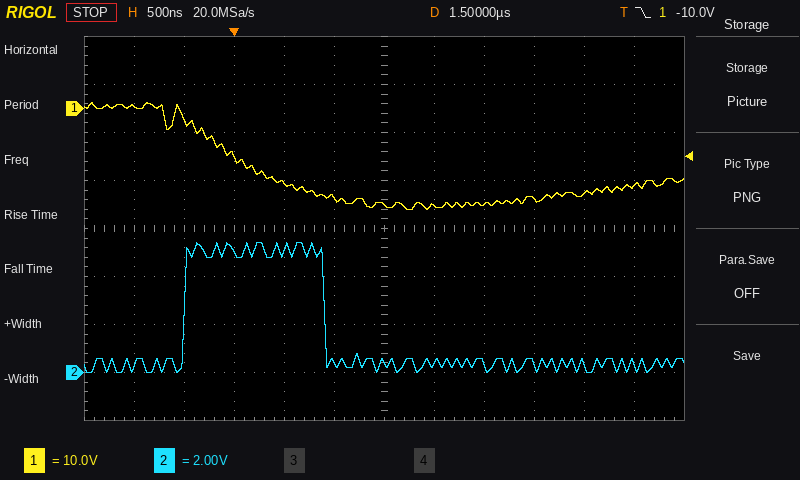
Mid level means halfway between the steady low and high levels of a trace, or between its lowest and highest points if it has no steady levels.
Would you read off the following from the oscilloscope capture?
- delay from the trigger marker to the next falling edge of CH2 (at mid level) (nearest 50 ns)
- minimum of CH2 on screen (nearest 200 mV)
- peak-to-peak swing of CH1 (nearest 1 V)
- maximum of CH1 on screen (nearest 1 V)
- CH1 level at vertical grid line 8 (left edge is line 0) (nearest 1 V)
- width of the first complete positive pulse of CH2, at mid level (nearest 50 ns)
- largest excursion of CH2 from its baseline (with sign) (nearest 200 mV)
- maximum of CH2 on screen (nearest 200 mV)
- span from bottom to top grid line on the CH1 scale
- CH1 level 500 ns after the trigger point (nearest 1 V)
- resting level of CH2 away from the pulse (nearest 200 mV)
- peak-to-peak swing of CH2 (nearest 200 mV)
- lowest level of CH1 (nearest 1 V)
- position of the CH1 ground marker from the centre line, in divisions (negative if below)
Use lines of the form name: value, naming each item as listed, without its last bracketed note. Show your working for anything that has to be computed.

delay from the trigger marker to the next falling edge of CH2 (at mid level): 900 ns
minimum of CH2 on screen: 0.0 V
peak-to-peak swing of CH1: 1 V − (-21 V) = 22 V
maximum of CH1 on screen: 1 V
CH1 level at vertical grid line 8 (left edge is line 0): -20 V
width of the first complete positive pulse of CH2, at mid level: 1.40 µs
largest excursion of CH2 from its baseline (with sign): 5.4 V − (400 mV) = +5.0 V
maximum of CH2 on screen: 5.4 V
span from bottom to top grid line on the CH1 scale: 80 V
CH1 level 500 ns after the trigger point: -16 V
resting level of CH2 away from the pulse: 400 mV
peak-to-peak swing of CH2: 5.4 V − (0.0 V) = 5.4 V
lowest level of CH1: -21 V
position of the CH1 ground marker from the centre line, in divisions: +2.5 div
